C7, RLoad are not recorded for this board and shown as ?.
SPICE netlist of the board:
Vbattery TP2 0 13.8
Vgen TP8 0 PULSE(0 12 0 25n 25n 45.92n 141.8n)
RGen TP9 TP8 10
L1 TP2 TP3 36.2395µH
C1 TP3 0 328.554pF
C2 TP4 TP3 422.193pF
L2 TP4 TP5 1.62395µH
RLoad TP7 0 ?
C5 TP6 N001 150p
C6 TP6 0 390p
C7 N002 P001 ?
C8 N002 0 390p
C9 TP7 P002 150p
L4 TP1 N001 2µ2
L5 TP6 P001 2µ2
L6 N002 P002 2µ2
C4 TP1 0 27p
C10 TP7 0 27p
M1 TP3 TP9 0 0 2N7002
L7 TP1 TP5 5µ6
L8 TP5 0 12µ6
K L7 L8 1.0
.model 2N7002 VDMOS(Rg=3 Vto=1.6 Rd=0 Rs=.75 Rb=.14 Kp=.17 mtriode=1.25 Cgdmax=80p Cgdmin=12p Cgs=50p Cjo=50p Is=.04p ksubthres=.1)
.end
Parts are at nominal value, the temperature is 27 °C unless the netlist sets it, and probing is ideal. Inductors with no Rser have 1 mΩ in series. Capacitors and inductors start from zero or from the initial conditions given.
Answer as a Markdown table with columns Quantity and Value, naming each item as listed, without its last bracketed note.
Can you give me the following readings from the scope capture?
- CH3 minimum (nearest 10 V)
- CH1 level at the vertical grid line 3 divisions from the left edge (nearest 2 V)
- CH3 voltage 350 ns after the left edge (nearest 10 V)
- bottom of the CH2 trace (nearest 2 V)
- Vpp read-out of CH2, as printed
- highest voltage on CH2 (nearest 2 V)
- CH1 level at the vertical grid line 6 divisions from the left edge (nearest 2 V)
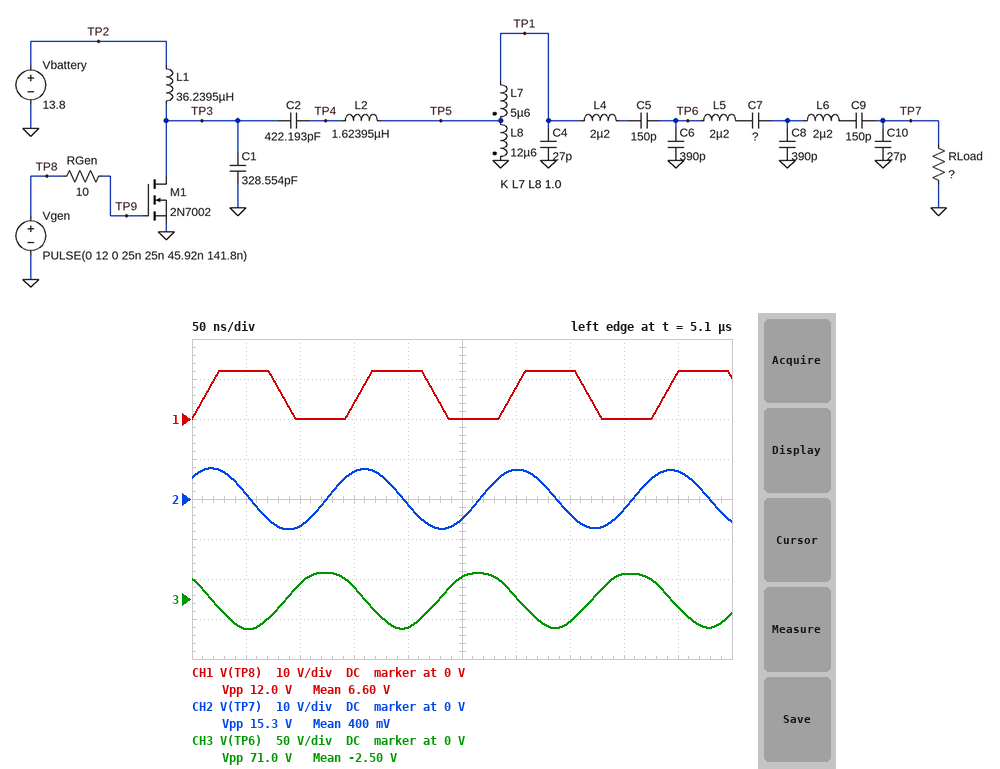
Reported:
| Quantity | Value |
|---|---|
| CH3 minimum | -40 V |
| CH1 level at the vertical grid line 3 divisions from the left edge | 4 V |
| CH3 voltage 350 ns after the left edge | -30 V |
| bottom of the CH2 trace | -8 V |
| Vpp read-out of CH2, as printed | 15.3 V |
| highest voltage on CH2 | 8 V |
| CH1 level at the vertical grid line 6 divisions from the left edge | 8 V |
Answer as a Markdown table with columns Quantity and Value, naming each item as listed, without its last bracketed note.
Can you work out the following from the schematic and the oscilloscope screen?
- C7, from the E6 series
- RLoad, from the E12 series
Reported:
| Quantity | Value |
|---|---|
| C7, from the E6 series | 680 pF |
| RLoad, from the E12 series | 15 Ω |
